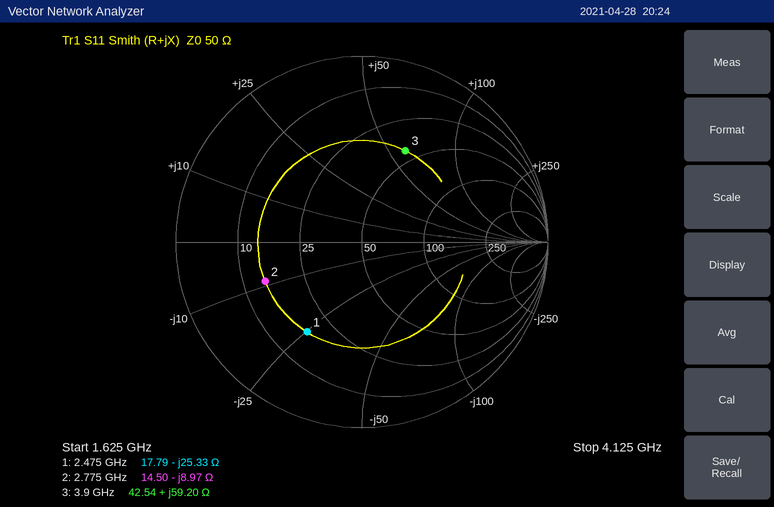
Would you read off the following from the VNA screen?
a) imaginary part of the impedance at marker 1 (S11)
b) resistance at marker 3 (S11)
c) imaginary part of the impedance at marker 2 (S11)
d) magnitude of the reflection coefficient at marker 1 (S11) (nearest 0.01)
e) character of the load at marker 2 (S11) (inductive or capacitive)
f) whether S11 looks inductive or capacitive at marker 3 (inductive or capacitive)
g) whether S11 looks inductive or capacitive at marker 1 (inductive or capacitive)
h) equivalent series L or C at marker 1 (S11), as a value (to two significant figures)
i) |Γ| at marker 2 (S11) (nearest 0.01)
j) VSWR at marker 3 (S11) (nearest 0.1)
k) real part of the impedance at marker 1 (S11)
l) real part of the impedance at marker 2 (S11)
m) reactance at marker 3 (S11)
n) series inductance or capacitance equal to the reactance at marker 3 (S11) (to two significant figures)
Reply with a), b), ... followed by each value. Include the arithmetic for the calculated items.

a) -25.33 Ω
b) 42.54 Ω
c) -8.97 Ω
d) 0.57
e) capacitive
f) inductive
g) capacitive
h) C = 1/(2π × 2.475 GHz × 25.33 Ω) ≈ 2.5 pF
i) 0.56
j) 3.4
k) 17.79 Ω
l) 14.50 Ω
m) +59.20 Ω
n) L = 59.2 Ω/(2π × 3.9 GHz) ≈ 2.4 nH
